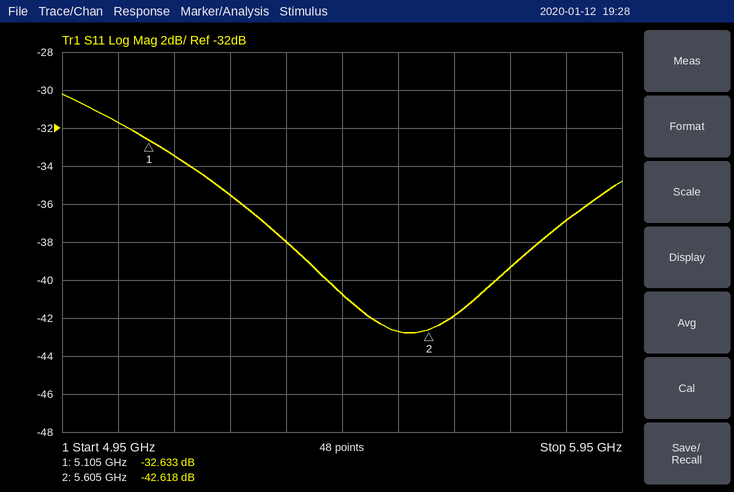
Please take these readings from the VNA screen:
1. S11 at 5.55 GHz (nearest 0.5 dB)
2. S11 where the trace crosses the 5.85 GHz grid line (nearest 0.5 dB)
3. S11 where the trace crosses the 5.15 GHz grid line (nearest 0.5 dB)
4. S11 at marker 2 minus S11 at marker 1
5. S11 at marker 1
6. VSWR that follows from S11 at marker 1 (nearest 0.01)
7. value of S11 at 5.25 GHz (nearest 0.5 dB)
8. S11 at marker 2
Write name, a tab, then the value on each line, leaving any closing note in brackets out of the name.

S11 at 5.55 GHz	-42.5 dB
S11 where the trace crosses the 5.85 GHz grid line	-37.0 dB
S11 where the trace crosses the 5.15 GHz grid line	-33.5 dB
S11 at marker 2 minus S11 at marker 1	-9.985 dB
S11 at marker 1	-32.633 dB
VSWR that follows from S11 at marker 1	1.05
value of S11 at 5.25 GHz	-35.5 dB
S11 at marker 2	-42.618 dB
